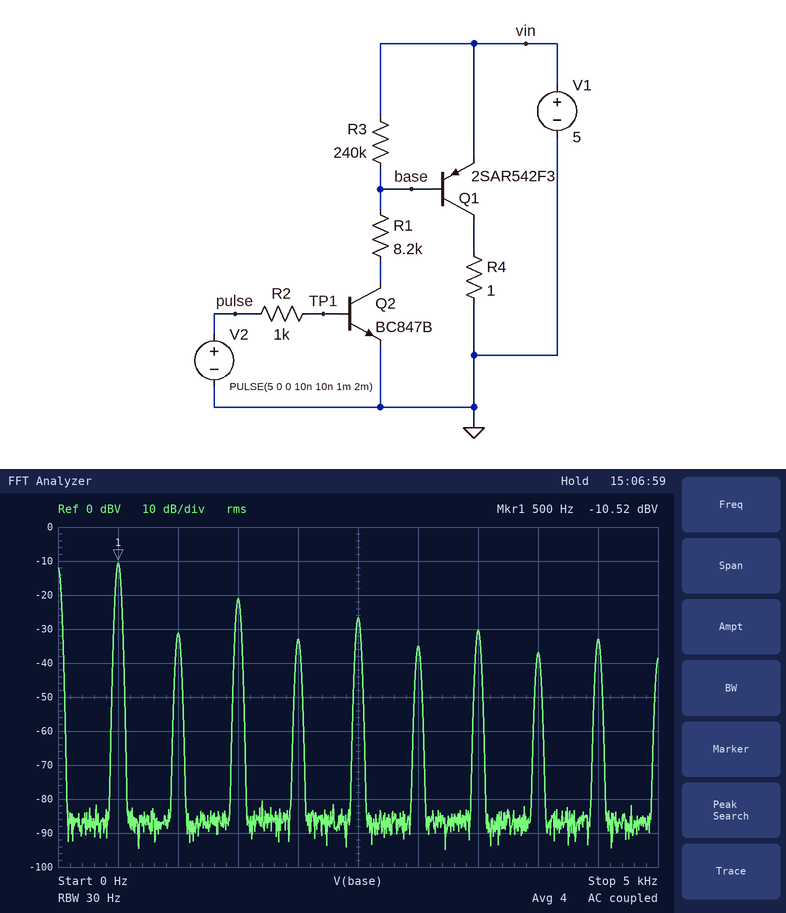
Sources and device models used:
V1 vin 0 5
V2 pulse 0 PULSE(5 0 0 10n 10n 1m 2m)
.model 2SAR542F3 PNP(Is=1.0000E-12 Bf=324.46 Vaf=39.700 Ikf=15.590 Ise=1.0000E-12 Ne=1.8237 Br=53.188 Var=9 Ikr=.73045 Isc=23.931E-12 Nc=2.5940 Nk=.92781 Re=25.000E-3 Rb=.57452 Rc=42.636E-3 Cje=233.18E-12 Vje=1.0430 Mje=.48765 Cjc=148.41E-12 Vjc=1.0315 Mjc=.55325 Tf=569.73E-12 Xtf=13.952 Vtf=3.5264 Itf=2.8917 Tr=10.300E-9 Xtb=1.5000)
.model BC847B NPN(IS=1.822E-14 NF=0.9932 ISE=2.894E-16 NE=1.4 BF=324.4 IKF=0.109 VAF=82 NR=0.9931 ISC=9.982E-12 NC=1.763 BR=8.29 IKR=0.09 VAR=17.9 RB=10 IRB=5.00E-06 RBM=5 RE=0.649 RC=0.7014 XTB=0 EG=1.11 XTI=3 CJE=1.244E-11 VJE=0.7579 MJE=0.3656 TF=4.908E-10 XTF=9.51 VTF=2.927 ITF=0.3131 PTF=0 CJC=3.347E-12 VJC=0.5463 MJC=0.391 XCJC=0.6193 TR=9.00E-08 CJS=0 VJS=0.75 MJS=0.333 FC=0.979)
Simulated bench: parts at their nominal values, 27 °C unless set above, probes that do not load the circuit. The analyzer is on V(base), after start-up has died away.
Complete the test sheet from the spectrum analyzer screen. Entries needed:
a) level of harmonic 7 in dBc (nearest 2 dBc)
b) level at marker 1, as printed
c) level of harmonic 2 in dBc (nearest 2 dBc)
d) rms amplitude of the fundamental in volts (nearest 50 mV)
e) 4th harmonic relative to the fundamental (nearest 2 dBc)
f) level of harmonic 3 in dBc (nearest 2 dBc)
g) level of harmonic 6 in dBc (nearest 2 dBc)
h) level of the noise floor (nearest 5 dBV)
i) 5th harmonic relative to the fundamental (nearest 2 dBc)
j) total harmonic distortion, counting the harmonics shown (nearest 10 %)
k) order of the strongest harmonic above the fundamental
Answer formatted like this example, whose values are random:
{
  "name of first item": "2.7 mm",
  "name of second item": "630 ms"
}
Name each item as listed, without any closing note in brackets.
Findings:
{
  "level of harmonic 7 in dBc": "-20 dBc",
  "level at marker 1, as printed": "-10.52 dBV",
  "level of harmonic 2 in dBc": "-20 dBc",
  "rms amplitude of the fundamental in volts": "300 mV",
  "4th harmonic relative to the fundamental": "-22 dBc",
  "level of harmonic 3 in dBc": "-10 dBc",
  "level of harmonic 6 in dBc": "-24 dBc",
  "level of the noise floor": "-85 dBV",
  "5th harmonic relative to the fundamental": "-16 dBc",
  "total harmonic distortion, counting the harmonics shown": "40 %",
  "order of the strongest harmonic above the fundamental": "3"
}
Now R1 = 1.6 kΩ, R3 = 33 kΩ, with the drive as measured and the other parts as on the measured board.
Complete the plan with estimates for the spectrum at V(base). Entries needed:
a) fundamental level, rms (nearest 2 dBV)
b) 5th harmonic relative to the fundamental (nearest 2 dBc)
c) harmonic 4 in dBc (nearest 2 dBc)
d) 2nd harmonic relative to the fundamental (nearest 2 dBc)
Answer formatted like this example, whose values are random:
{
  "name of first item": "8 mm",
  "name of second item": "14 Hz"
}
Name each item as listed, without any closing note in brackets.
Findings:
{
  "fundamental level, rms": "-10 dBV",
  "5th harmonic relative to the fundamental": "-14 dBc",
  "harmonic 4 in dBc": "-36 dBc",
  "2nd harmonic relative to the fundamental": "-36 dBc"
}
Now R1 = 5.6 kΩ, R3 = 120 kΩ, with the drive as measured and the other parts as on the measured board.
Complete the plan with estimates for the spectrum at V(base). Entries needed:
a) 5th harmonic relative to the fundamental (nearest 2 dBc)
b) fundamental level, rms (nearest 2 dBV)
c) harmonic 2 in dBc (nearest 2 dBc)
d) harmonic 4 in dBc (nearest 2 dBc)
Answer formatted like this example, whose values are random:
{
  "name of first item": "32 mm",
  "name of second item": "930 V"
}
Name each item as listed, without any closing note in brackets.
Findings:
{
  "5th harmonic relative to the fundamental": "-14 dBc",
  "fundamental level, rms": "-10 dBV",
  "harmonic 2 in dBc": "-26 dBc",
  "harmonic 4 in dBc": "-26 dBc"
}
